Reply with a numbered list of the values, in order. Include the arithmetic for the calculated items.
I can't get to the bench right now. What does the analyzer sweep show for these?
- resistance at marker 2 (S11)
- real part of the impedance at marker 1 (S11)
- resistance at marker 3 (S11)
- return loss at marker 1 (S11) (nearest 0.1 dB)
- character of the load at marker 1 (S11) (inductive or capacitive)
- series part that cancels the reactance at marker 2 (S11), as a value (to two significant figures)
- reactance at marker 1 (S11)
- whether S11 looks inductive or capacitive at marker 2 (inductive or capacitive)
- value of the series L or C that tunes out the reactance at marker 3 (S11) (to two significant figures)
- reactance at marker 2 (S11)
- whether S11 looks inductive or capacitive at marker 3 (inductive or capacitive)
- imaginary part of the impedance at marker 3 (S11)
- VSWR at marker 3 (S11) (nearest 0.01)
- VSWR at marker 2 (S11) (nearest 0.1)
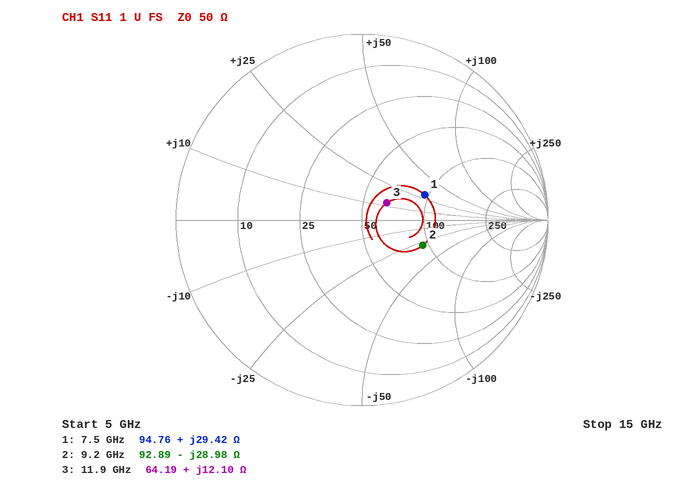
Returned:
1. 92.89 Ω
2. 94.76 Ω
3. 64.19 Ω
4. 8.8 dB
5. inductive
6. L = 28.98 Ω/(2π × 9.2 GHz) ≈ 501 pH, so 500 pH to two significant figures
7. +29.42 Ω
8. capacitive
9. C = 1/(2π × 11.9 GHz × 12.1 Ω) ≈ 1.1 pF
10. -28.98 Ω
11. inductive
12. +12.10 Ω
13. 1.39
14. 2.1
